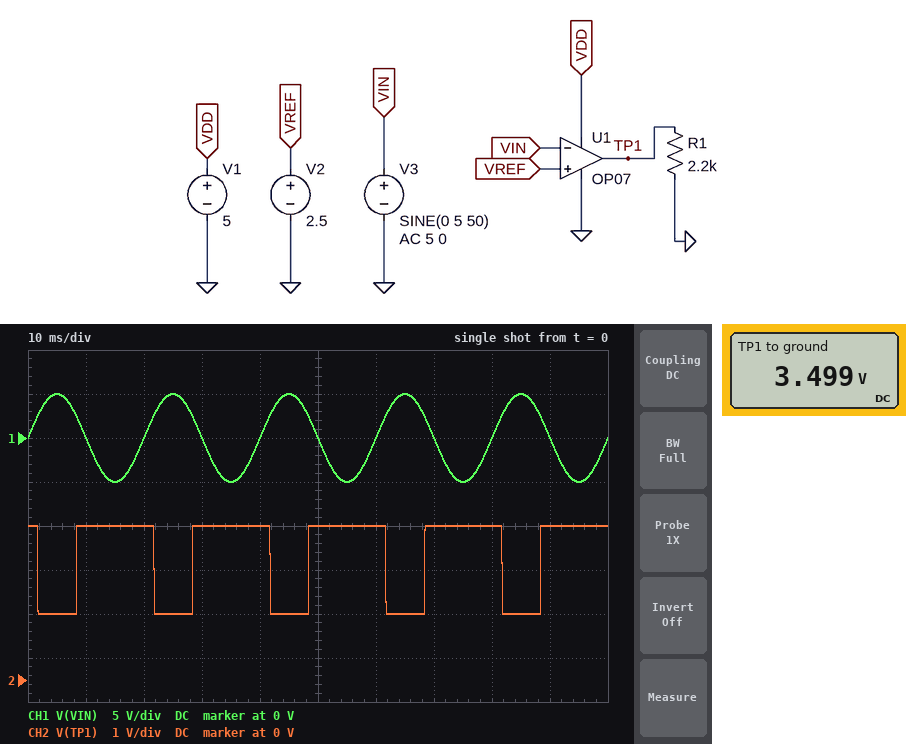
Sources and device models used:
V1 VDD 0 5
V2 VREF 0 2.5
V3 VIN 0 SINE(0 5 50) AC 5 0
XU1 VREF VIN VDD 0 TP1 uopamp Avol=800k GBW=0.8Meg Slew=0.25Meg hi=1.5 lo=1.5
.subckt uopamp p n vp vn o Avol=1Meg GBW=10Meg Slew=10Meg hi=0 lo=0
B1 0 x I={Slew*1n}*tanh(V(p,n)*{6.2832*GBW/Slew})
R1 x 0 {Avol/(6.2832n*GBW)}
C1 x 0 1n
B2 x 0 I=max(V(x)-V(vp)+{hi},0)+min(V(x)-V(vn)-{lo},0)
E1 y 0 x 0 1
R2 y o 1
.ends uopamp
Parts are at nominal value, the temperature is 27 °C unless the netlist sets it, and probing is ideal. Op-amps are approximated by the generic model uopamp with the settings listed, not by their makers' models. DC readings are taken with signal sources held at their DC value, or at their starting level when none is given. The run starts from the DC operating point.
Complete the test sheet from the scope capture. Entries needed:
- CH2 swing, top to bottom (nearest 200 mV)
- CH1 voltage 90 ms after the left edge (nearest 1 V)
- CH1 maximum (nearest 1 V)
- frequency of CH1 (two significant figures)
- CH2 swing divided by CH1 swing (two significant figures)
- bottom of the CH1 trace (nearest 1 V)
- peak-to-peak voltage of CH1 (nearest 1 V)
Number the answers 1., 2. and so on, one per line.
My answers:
1. 2.0 V
2. 0 V
3. 5 V
4. 50 Hz
5. 0.20
6. -5 V
7. 10 V
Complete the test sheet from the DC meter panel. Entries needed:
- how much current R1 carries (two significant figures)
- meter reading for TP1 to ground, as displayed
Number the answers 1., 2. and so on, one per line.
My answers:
1. 1.6 mA
2. 3.499 V
